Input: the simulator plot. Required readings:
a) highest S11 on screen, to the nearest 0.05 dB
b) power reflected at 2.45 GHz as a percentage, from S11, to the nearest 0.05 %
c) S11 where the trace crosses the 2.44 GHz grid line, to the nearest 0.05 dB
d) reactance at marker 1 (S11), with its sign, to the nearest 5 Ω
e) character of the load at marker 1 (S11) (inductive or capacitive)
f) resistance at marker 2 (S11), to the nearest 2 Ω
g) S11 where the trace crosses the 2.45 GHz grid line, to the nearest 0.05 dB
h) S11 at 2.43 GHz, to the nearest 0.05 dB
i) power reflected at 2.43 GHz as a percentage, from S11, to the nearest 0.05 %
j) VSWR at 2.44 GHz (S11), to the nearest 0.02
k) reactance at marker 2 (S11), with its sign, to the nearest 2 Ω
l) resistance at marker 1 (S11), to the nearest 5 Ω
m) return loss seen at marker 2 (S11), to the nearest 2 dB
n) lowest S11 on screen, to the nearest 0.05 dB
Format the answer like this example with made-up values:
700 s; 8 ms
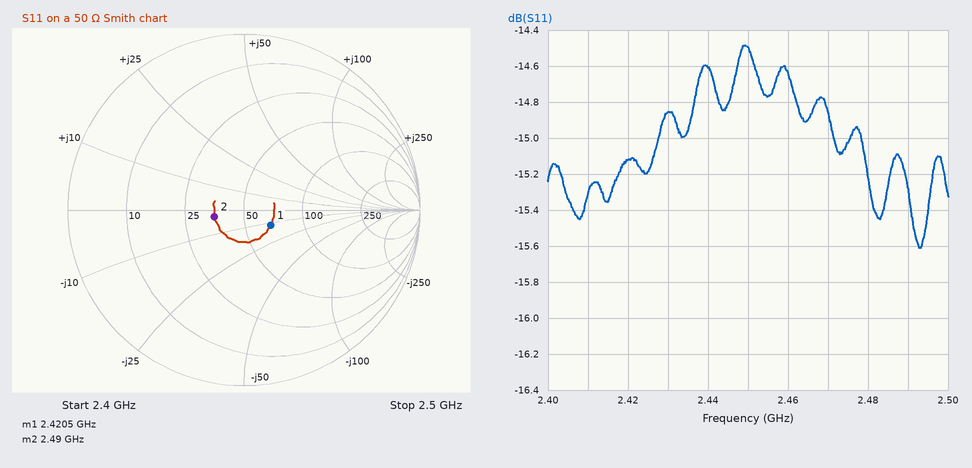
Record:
-14.50 dB; 3.55 %; -14.60 dB; -10 Ω; capacitive; 36 Ω; -14.50 dB; -14.85 dB; 3.25 %; 1.46; -2 Ω; 65 Ω; 16 dB; -15.60 dB
